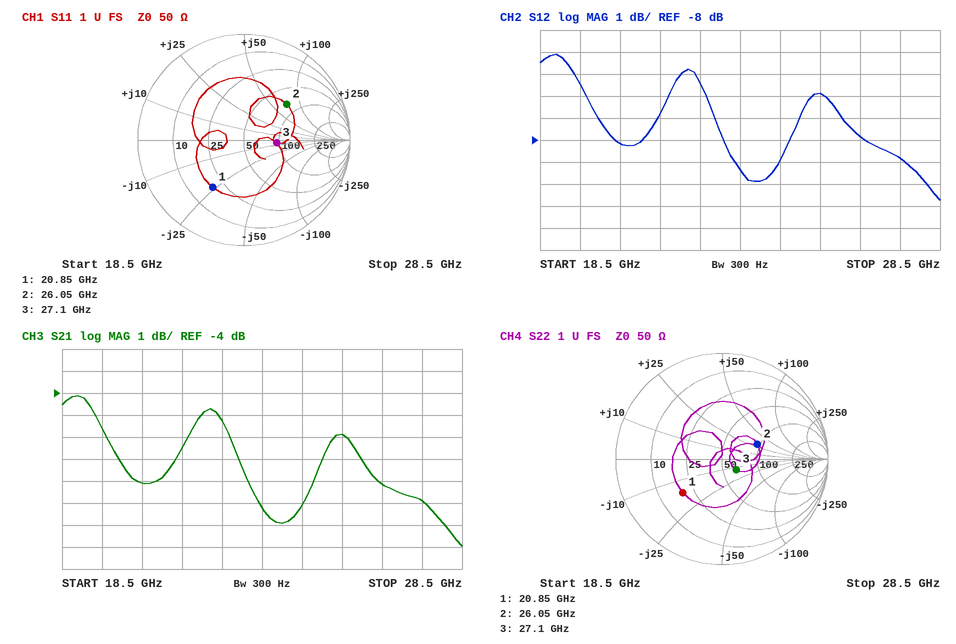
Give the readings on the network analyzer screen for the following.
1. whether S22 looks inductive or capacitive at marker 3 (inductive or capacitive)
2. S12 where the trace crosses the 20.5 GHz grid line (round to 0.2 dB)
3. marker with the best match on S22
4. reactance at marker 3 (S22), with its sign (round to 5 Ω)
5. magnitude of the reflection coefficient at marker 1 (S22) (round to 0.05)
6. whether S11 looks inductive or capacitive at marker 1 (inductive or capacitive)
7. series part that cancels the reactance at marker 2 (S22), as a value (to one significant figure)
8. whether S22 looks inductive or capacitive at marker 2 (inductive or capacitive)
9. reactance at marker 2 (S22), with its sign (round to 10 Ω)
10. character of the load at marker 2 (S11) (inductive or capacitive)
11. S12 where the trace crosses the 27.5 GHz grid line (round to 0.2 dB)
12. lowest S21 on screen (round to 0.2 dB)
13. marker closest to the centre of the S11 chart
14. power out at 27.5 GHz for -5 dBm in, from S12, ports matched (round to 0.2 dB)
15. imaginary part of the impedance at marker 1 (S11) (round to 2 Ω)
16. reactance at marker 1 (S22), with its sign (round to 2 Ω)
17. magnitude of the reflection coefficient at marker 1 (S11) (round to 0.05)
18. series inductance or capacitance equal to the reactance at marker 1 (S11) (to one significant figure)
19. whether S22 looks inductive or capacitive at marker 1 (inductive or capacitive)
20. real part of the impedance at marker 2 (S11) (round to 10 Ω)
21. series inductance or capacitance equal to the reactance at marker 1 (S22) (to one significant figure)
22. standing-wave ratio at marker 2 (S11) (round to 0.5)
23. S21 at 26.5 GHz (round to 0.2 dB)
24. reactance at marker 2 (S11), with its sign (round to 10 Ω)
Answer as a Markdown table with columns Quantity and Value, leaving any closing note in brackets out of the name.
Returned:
| Quantity | Value |
|---|---|
| whether S22 looks inductive or capacitive at marker 3 | capacitive |
| S12 where the trace crosses the 20.5 GHz grid line | -8.2 dB |
| marker with the best match on S22 | marker 3 |
| reactance at marker 3 (S22), with its sign | -15 Ω |
| magnitude of the reflection coefficient at marker 1 (S22) | 0.50 |
| whether S11 looks inductive or capacitive at marker 1 | capacitive |
| series part that cancels the reactance at marker 2 (S22), as a value | 200 fF |
| whether S22 looks inductive or capacitive at marker 2 | inductive |
| reactance at marker 2 (S22), with its sign | +30 Ω |
| character of the load at marker 2 (S11) | inductive |
| S12 where the trace crosses the 27.5 GHz grid line | -8.8 dB |
| lowest S21 on screen | -11.0 dB |
| marker closest to the centre of the S11 chart | marker 3 |
| power out at 27.5 GHz for -5 dBm in, from S12, ports matched | -13.8 dBm |
| imaginary part of the impedance at marker 1 (S11) | -24 Ω |
| reactance at marker 1 (S22), with its sign | -16 Ω |
| magnitude of the reflection coefficient at marker 1 (S11) | 0.55 |
| series inductance or capacitance equal to the reactance at marker 1 (S11) | 300 fF |
| whether S22 looks inductive or capacitive at marker 1 | capacitive |
| real part of the impedance at marker 2 (S11) | 80 Ω |
| series inductance or capacitance equal to the reactance at marker 1 (S22) | 500 fF |
| standing-wave ratio at marker 2 (S11) | 3.0 |
| S21 at 26.5 GHz | -8.2 dB |
| reactance at marker 2 (S11), with its sign | +70 Ω |
